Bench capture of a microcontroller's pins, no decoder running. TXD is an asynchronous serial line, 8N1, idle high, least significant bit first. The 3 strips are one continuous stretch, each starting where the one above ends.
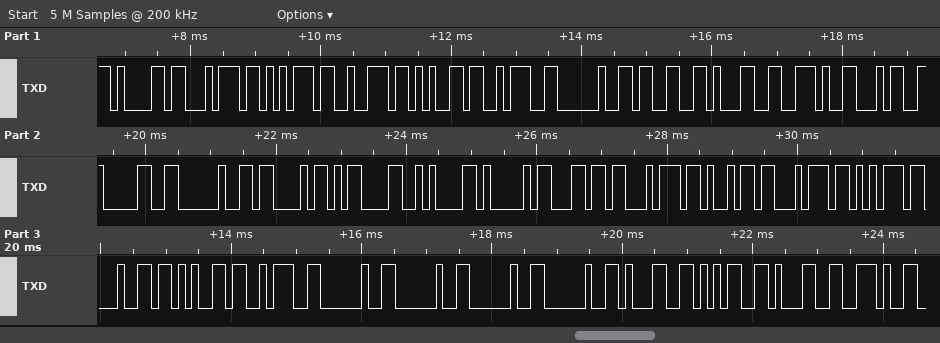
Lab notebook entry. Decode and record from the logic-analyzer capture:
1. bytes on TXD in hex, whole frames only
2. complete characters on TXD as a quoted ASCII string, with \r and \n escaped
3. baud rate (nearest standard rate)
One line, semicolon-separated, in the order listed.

61 74 75 72 65 3A 20 33 31 2E 34 30 20 43 0D 0A 41 6C 74 69 74 75 64 65 3A 20 20 20 20 31 35 31 2E; "ature: 31.40 C\r\nAltitude:    151."; 9600 baud
